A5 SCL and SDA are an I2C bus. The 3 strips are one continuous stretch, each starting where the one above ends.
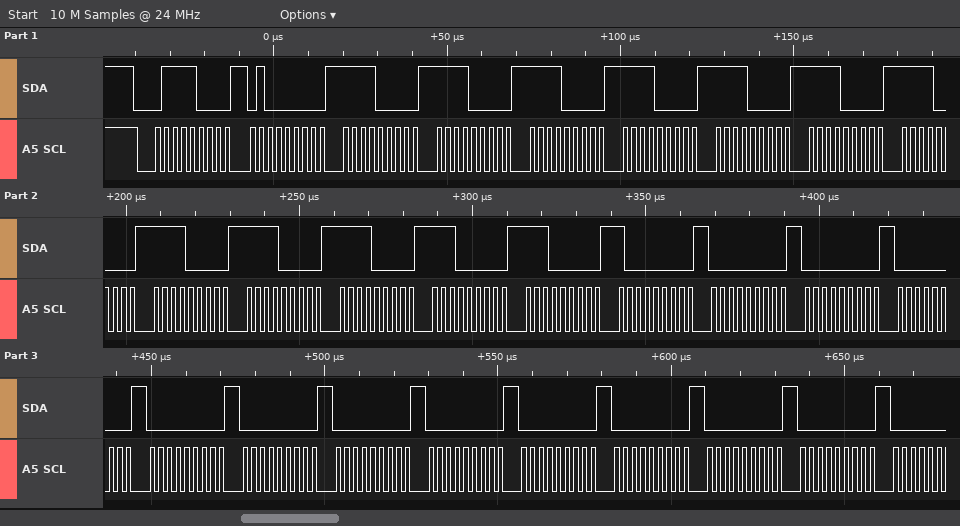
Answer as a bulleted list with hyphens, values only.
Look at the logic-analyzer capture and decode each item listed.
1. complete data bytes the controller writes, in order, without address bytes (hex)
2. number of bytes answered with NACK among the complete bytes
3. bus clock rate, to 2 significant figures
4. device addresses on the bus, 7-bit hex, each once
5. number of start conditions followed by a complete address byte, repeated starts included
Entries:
- 40 F0 F0 F0 F0 F0 F0 F0 F0 F0 F0 E0 E0 80 00 00 00 00 00 00 00 00 00 00 00
- 0
- 400 kHz
- 0x3C
- 1
